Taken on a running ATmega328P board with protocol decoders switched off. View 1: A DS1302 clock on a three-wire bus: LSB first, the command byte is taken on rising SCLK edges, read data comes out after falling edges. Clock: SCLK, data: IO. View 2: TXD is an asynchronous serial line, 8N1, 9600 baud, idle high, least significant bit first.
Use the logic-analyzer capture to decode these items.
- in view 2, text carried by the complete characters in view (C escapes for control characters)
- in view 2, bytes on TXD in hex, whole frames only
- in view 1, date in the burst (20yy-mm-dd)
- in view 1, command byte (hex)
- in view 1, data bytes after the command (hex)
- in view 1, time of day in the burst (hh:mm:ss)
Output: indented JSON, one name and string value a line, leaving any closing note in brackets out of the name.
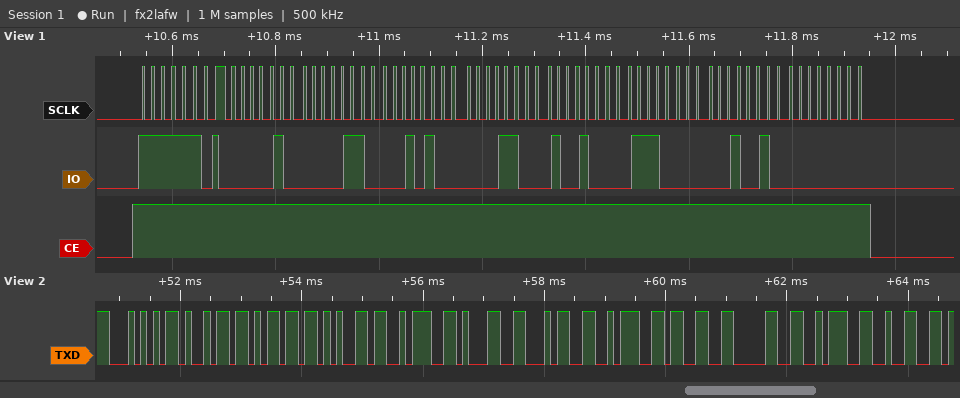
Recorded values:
{
  "in view 2, text carried by the complete characters in view": "\"Time:14:30:2\"",
  "in view 2, bytes on TXD in hex, whole frames only": "54 69 6D 65 3A 31 34 3A 33 30 3A 32",
  "in view 1, date in the burst": "2024-09-18",
  "in view 1, command byte": "0xBF",
  "in view 1, data bytes after the command": "20 30 14 18 09 07 24 00",
  "in view 1, time of day in the burst": "14:30:20"
}
